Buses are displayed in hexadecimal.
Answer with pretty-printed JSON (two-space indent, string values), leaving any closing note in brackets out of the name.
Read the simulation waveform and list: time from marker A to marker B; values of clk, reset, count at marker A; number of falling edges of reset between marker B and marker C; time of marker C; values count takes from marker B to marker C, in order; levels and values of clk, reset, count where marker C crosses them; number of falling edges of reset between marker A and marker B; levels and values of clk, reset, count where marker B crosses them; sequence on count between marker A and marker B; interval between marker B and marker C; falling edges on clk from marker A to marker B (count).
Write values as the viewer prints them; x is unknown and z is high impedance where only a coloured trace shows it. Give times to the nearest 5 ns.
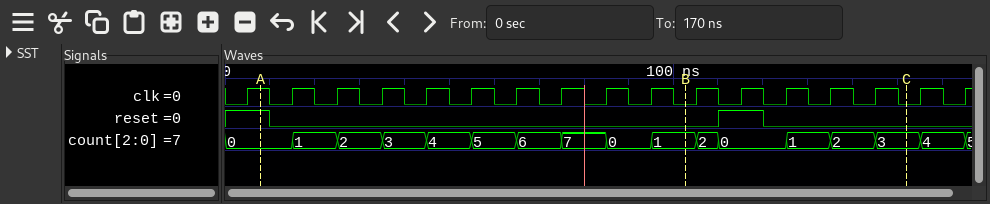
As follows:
{
  "time from marker A to marker B": "95 ns",
  "values of clk, reset, count at marker A": "clk=1, reset=1, count=0",
  "number of falling edges of reset between marker B and marker C": "1",
  "time of marker C": "150 ns",
  "values count takes from marker B to marker C, in order": "1, 2, 0, 1, 2, 3",
  "levels and values of clk, reset, count where marker C crosses them": "clk=0, reset=0, count=3",
  "number of falling edges of reset between marker A and marker B": "1",
  "levels and values of clk, reset, count where marker B crosses them": "clk=0, reset=0, count=1",
  "sequence on count between marker A and marker B": "0, 1, 2, 3, 4, 5, 6, 7, 0, 1",
  "interval between marker B and marker C": "50 ns",
  "falling edges on clk from marker A to marker B": "10"
}
